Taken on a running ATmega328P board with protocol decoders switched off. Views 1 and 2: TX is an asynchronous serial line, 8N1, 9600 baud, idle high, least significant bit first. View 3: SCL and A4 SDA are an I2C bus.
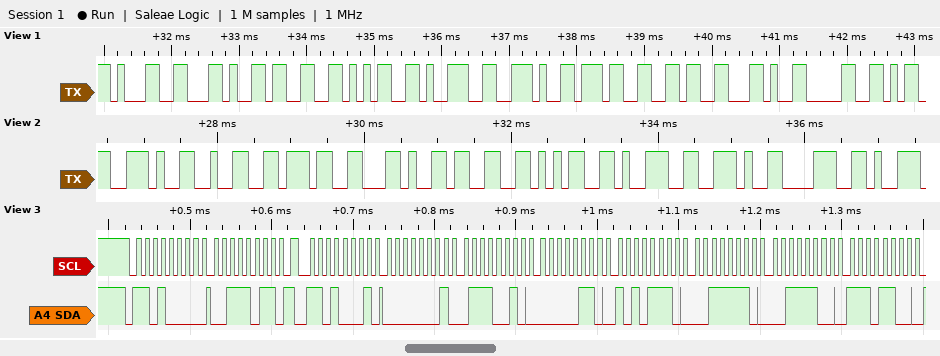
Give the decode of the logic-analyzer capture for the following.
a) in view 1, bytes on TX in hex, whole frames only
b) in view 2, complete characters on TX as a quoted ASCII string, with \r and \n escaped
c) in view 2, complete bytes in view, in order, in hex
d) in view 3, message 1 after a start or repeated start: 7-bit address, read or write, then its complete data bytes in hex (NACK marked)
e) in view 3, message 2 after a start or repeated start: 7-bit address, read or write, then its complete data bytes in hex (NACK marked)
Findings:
0x31 0x2C 0x33 0x35 0x39 0x2E 0x37 0x36 0x2C 0x30
".27,359.8"
2E 32 37 2C 33 35 39 2E 38
0x68 write: 3B
0x68 read: 01 72 06 AE 3E 3C EC
